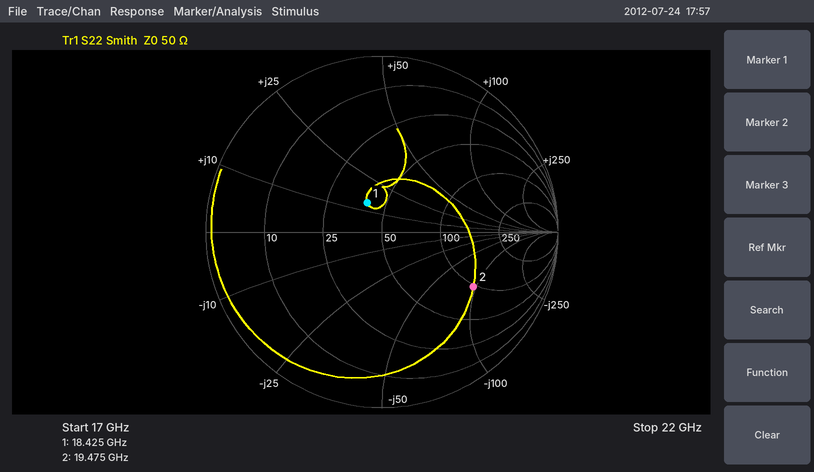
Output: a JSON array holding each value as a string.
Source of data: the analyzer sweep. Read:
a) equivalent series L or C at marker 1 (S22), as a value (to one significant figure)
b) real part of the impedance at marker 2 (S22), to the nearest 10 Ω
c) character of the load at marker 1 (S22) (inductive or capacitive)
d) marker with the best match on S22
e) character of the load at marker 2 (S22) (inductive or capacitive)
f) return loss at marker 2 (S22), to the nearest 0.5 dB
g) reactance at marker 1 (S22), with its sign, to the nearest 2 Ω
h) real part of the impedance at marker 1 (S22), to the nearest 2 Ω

["100 pH", "100 Ω", "inductive", "marker 1", "capacitive", "4.5 dB", "+14 Ω", "40 Ω"]
